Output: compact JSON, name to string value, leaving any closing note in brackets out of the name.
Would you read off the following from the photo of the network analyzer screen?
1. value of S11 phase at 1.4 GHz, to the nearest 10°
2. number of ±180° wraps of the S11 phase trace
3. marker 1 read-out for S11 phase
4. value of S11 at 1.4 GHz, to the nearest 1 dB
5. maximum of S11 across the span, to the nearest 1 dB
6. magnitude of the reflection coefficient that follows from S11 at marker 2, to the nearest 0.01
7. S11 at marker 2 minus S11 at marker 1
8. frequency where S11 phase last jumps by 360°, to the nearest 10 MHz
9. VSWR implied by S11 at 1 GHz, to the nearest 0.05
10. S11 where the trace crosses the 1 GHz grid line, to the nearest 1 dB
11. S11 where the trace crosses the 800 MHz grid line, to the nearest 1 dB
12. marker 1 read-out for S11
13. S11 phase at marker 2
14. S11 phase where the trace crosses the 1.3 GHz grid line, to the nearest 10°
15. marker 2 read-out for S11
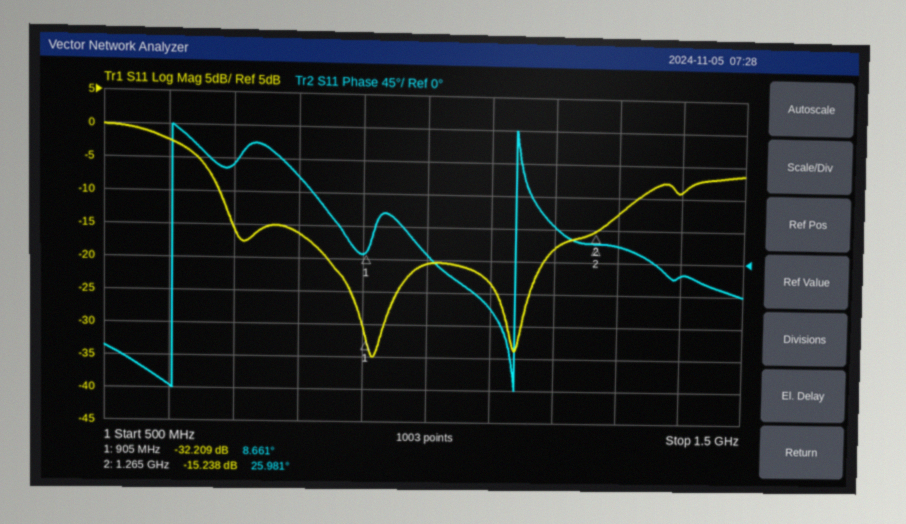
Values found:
{"value of S11 phase at 1.4 GHz, to the nearest 10°": "-20°", "number of ±180° wraps of the S11 phase trace": "2", "marker 1 read-out for S11 phase": "8.661°", "value of S11 at 1.4 GHz, to the nearest 1 dB": "-9 dB", "maximum of S11 across the span, to the nearest 1 dB": "0 dB", "magnitude of the reflection coefficient that follows from S11 at marker 2, to the nearest 0.01": "0.17", "S11 at marker 2 minus S11 at marker 1": "16.971 dB", "frequency where S11 phase last jumps by 360°, to the nearest 10 MHz": "1.14 GHz", "VSWR implied by S11 at 1 GHz, to the nearest 0.05": "1.20", "S11 where the trace crosses the 1 GHz grid line, to the nearest 1 dB": "-21 dB", "S11 where the trace crosses the 800 MHz grid line, to the nearest 1 dB": "-16 dB", "marker 1 read-out for S11": "-32.209 dB", "S11 phase at marker 2": "25.981°", "S11 phase where the trace crosses the 1.3 GHz grid line, to the nearest 10°": "20°", "marker 2 read-out for S11": "-15.238 dB"}
